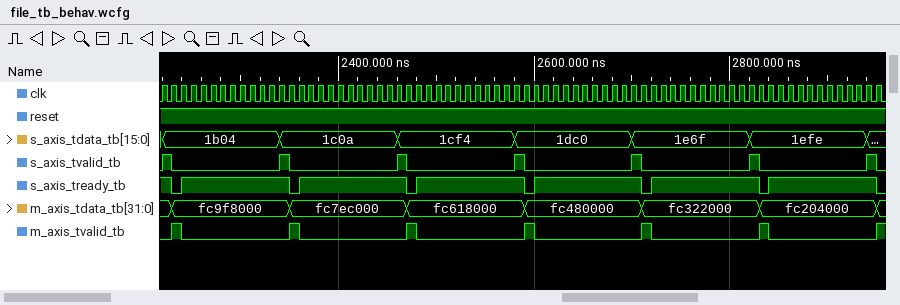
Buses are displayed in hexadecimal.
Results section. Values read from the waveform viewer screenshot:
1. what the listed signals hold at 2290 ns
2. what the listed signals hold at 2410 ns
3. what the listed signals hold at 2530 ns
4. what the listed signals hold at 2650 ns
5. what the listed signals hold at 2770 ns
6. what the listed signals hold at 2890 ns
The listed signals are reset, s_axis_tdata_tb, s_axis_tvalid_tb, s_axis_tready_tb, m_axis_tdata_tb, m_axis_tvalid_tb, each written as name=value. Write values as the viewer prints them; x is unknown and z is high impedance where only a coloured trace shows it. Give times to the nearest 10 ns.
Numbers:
reset=1, s_axis_tdata_tb=1b04, s_axis_tvalid_tb=0, s_axis_tready_tb=1, m_axis_tdata_tb=fc9f8000, m_axis_tvalid_tb=0
reset=1, s_axis_tdata_tb=1c0a, s_axis_tvalid_tb=0, s_axis_tready_tb=1, m_axis_tdata_tb=fc7ec000, m_axis_tvalid_tb=0
reset=1, s_axis_tdata_tb=1cf4, s_axis_tvalid_tb=0, s_axis_tready_tb=1, m_axis_tdata_tb=fc618000, m_axis_tvalid_tb=0
reset=1, s_axis_tdata_tb=1dc0, s_axis_tvalid_tb=0, s_axis_tready_tb=1, m_axis_tdata_tb=fc480000, m_axis_tvalid_tb=0
reset=1, s_axis_tdata_tb=1e6f, s_axis_tvalid_tb=0, s_axis_tready_tb=1, m_axis_tdata_tb=fc322000, m_axis_tvalid_tb=0
reset=1, s_axis_tdata_tb=1efe, s_axis_tvalid_tb=0, s_axis_tready_tb=1, m_axis_tdata_tb=fc204000, m_axis_tvalid_tb=0
